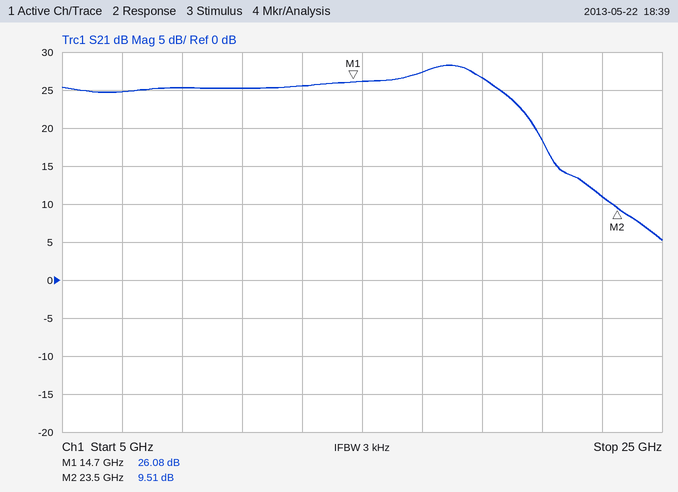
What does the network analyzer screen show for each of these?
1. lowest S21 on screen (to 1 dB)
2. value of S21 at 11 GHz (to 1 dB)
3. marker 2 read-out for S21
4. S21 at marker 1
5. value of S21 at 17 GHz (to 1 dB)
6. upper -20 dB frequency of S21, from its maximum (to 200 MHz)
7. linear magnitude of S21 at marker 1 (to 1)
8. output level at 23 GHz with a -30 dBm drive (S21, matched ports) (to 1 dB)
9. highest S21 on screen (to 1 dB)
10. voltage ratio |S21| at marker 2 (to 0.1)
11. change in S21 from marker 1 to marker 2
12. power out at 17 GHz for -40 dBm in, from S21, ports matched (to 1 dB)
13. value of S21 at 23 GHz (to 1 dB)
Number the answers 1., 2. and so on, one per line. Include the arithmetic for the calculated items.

1. 5 dB
2. 25 dB
3. 9.51 dB
4. 26.08 dB
5. 27 dB
6. 24.0 GHz
7. 10^(26.08/20) ≈ 20
8. -30 dBm + (11 dB) = -19 dBm
9. 28 dB
10. 10^(9.51/20) ≈ 3.0
11. 9.51 − (26.08) = -16.57 dB
12. -40 dBm + (27 dB) = -13 dBm
13. 11 dB
